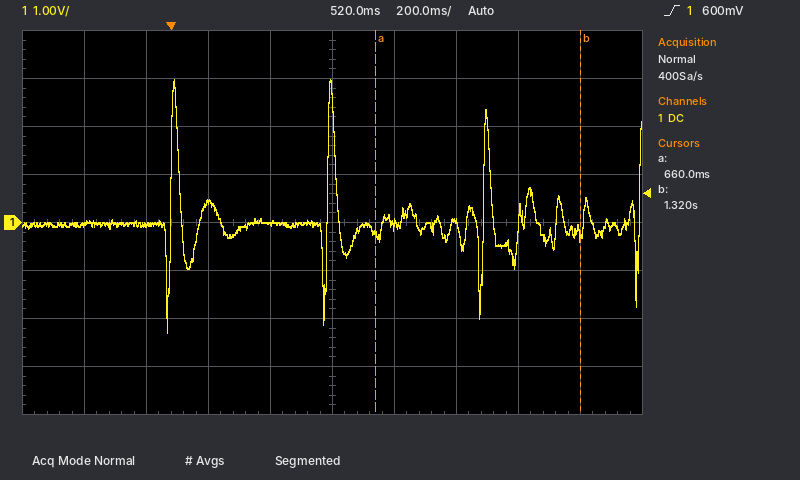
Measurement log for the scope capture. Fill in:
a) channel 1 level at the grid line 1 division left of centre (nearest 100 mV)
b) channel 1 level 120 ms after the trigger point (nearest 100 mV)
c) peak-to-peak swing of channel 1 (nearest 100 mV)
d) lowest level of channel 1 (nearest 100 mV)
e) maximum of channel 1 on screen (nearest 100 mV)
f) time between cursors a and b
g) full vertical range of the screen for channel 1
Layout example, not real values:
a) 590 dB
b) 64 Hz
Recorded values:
a) 0.0 V
b) 400 mV
c) 5.3 V
d) -2.3 V
e) 3.0 V
f) 660 ms
g) 8 V
